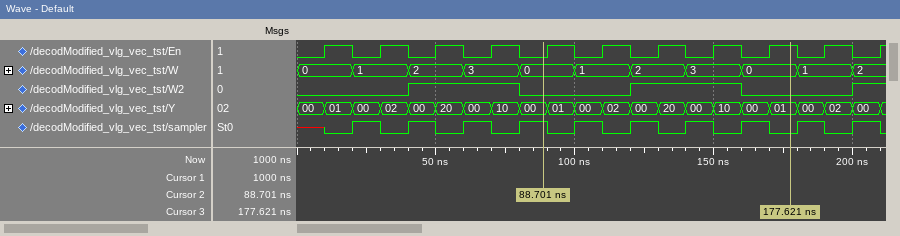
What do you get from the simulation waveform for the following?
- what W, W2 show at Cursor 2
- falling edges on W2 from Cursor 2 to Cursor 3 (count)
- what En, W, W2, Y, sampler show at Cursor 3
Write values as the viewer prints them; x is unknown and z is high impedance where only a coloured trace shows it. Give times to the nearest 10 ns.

W=0, W2=0
1
En=1, W=0, W2=0, Y=01, sampler=0
